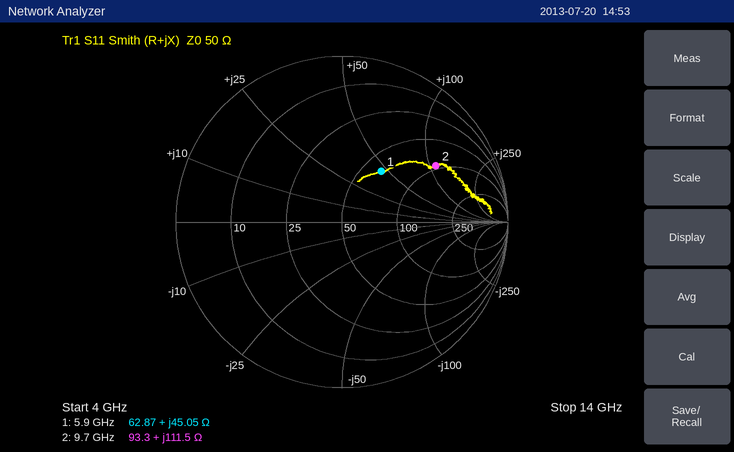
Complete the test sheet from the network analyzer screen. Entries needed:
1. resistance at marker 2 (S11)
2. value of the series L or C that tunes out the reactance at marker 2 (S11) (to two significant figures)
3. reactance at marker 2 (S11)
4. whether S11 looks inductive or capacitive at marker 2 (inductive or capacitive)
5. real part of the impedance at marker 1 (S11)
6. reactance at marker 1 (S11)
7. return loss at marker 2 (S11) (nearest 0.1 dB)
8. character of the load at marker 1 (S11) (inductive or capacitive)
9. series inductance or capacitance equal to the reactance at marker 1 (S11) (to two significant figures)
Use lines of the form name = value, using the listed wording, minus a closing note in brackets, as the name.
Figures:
resistance at marker 2 = 93.3 Ω
value of the series L or C that tunes out the reactance at marker 2 (S11) = 150 fF
reactance at marker 2 = +111.5 Ω
whether S11 looks inductive or capacitive at marker 2 = inductive
real part of the impedance at marker 1 = 62.87 Ω
reactance at marker 1 = +45.05 Ω
return loss at marker 2 (S11) = 3.6 dB
character of the load at marker 1 (S11) = inductive
series inductance or capacitance equal to the reactance at marker 1 (S11) = 1.2 nH
